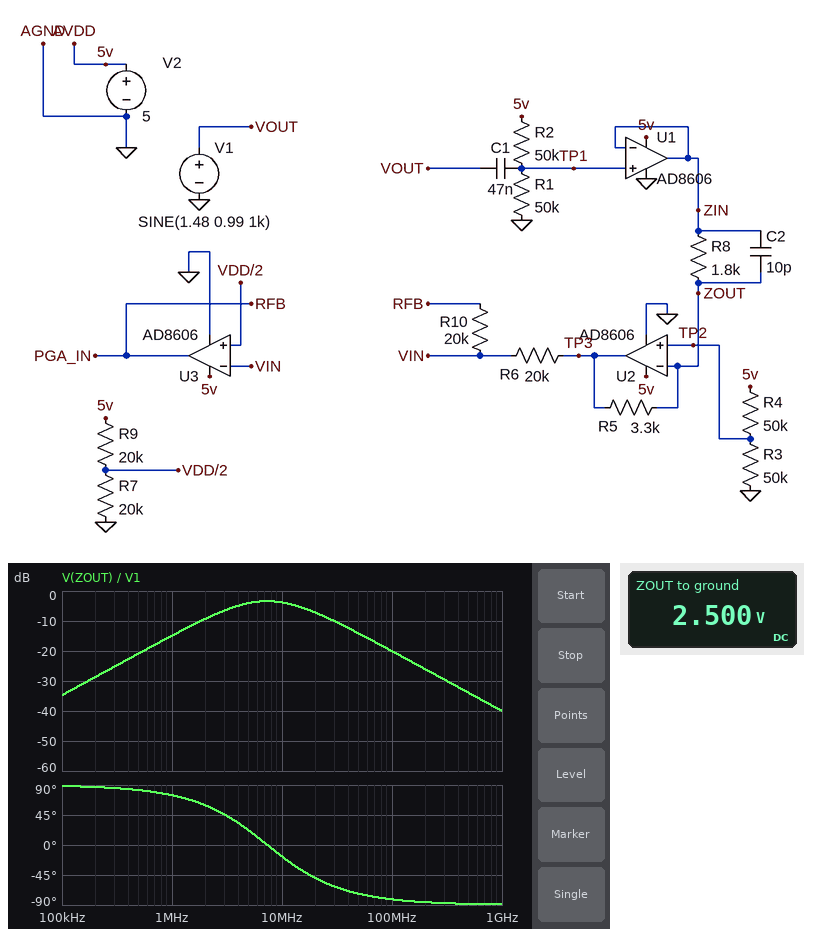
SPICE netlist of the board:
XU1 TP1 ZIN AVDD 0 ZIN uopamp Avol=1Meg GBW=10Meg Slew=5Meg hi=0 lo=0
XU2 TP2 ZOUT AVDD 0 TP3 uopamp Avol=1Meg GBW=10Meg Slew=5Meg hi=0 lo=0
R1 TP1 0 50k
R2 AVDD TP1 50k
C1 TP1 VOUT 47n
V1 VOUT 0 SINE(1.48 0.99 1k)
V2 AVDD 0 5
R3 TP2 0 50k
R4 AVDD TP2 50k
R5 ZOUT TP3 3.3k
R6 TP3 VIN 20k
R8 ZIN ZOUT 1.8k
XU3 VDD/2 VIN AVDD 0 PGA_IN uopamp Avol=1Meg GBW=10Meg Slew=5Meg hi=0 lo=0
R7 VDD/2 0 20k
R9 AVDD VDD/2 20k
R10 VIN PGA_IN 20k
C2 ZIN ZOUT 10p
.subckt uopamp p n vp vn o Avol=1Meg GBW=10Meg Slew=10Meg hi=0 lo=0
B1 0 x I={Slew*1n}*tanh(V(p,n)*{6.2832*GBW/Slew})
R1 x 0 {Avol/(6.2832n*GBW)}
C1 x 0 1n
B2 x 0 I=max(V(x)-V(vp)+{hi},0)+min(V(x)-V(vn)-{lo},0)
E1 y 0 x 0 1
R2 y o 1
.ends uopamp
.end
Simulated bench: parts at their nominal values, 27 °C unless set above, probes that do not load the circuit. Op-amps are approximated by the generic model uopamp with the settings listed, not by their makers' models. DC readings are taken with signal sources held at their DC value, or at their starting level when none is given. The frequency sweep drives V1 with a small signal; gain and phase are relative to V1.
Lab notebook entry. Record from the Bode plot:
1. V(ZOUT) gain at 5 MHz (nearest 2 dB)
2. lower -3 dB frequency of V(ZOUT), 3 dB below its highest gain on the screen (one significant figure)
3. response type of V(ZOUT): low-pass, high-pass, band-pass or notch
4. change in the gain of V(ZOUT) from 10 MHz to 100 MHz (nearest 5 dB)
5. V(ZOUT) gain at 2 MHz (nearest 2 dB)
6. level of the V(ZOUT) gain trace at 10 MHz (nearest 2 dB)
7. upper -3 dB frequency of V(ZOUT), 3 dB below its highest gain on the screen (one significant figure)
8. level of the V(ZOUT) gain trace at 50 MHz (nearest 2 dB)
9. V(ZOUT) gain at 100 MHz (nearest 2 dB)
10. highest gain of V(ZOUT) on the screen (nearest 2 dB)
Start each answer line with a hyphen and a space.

- -4 dB
- 3 MHz
- band-pass
- -15 dB
- -10 dB
- -4 dB
- 20 MHz
- -14 dB
- -20 dB
- -4 dB
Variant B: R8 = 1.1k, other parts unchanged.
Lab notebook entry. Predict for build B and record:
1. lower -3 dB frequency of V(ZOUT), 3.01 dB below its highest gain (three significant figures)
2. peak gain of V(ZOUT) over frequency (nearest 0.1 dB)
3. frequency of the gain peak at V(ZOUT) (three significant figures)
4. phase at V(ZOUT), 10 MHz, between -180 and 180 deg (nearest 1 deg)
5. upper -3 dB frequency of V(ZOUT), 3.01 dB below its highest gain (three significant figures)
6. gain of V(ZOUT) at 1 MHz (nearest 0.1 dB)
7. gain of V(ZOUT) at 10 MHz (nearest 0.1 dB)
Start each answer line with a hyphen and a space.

- 2.01 MHz
- -3.2 dB
- 5.63 MHz
- -25 deg
- 16.1 MHz
- -11.0 dB
- -4.1 dB
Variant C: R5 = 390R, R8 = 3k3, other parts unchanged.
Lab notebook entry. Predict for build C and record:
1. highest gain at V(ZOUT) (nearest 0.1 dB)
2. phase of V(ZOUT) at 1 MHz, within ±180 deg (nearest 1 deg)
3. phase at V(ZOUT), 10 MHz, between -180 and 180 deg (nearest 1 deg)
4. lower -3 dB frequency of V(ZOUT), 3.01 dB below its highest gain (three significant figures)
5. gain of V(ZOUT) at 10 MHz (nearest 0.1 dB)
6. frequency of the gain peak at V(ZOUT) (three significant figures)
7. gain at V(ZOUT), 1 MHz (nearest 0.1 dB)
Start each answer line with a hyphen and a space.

- -13.8 dB
- 90 deg
- 53 deg
- 10.1 MHz
- -16.9 dB
- 23.3 MHz
- -38.4 dB
